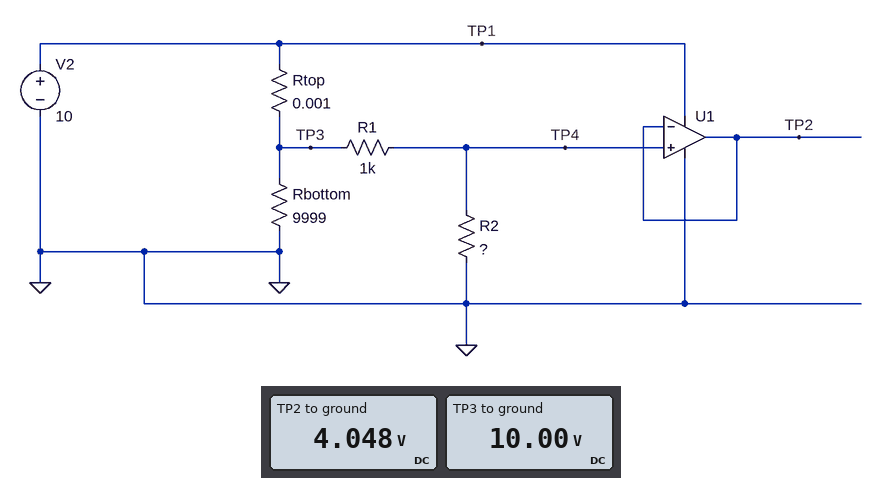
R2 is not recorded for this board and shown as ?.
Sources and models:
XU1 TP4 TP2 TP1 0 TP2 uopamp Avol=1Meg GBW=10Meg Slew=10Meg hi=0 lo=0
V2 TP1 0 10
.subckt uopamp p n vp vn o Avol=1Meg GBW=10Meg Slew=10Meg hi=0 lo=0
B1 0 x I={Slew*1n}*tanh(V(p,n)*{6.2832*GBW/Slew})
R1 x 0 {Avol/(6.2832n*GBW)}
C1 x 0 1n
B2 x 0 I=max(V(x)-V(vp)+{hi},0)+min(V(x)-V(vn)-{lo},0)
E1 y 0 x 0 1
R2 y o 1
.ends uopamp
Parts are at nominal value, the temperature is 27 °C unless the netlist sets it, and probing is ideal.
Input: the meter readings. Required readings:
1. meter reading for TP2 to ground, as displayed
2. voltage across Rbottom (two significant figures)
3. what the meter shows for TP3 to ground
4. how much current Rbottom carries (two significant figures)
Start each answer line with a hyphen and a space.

- 4.048 V
- 10 V
- 10.00 V
- 1.0 mA
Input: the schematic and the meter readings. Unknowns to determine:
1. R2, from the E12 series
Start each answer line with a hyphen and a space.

- 680 Ω
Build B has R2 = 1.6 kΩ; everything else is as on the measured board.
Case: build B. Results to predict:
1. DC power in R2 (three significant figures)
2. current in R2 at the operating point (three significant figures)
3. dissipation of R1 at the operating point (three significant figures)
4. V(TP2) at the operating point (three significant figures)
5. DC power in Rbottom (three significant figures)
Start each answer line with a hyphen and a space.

- 23.7 mW
- 3.85 mA
- 14.8 mW
- 6.15 V
- 10.0 mW
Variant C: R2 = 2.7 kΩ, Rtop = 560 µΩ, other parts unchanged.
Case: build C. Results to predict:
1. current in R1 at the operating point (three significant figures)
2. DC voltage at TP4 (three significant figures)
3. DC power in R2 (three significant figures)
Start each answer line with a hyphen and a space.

- 2.70 mA
- 7.30 V
- 19.7 mW
